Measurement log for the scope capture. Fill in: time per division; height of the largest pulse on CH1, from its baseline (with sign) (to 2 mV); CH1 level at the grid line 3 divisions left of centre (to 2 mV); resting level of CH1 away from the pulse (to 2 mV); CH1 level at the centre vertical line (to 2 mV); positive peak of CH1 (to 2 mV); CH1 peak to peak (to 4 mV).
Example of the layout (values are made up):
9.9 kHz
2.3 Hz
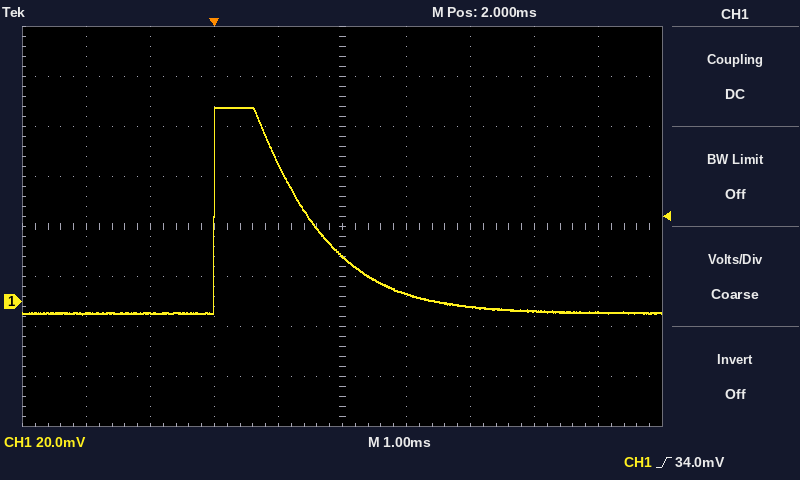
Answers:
1 ms
+82 mV
-4 mV
-4 mV
18 mV
78 mV
84 mV
